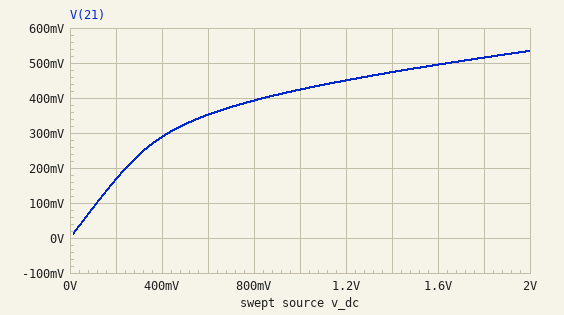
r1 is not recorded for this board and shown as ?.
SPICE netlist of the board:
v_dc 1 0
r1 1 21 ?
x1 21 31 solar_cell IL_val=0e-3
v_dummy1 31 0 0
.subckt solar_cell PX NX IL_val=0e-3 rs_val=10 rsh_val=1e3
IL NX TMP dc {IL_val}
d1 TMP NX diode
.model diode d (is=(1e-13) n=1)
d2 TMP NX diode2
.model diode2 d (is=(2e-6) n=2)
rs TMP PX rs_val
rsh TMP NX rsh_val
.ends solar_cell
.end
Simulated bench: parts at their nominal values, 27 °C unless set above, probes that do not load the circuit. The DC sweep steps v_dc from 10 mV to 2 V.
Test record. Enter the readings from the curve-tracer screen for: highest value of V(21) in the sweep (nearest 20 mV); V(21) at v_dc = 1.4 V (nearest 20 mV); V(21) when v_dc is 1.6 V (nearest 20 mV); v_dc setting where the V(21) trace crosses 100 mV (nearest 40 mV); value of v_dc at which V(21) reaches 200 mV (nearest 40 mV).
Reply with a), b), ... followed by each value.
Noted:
a) 540 mV
b) 480 mV
c) 500 mV
d) 120 mV
e) 240 mV
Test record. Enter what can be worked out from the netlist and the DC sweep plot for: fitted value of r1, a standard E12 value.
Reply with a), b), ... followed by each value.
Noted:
a) 150 Ω
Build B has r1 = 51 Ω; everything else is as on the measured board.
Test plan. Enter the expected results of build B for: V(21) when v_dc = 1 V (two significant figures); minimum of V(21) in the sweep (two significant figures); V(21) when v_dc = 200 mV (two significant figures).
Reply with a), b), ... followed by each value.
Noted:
a) 530 mV
b) 9.5 mV
c) 190 mV
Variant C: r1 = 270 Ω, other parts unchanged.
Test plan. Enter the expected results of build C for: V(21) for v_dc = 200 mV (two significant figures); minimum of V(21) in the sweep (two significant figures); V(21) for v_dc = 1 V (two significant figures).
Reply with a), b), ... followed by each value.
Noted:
a) 150 mV
b) 7.8 mV
c) 380 mV
